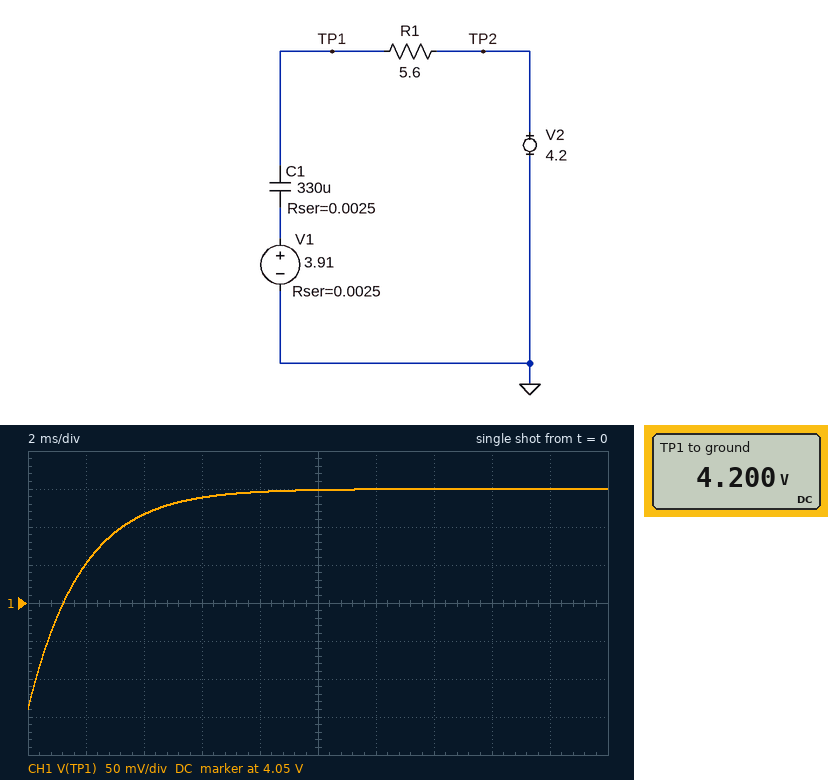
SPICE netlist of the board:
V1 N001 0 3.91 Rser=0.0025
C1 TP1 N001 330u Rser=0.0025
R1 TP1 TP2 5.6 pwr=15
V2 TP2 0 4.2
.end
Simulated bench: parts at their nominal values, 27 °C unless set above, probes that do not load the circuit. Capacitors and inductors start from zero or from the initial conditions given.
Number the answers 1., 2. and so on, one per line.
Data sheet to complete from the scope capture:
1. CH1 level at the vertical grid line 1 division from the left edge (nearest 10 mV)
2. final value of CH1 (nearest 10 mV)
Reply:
1. 4.10 V
2. 4.20 V
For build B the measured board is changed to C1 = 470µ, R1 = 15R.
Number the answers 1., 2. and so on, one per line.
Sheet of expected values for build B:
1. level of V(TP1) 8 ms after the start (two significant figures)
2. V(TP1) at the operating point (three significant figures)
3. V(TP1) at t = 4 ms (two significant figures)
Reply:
1. 4.1 V
2. 4.20 V
3. 4.0 V
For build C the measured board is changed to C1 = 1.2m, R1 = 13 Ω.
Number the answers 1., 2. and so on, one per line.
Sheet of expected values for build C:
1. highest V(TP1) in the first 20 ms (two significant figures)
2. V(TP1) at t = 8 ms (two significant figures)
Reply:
1. 4.1 V
2. 4.0 V
